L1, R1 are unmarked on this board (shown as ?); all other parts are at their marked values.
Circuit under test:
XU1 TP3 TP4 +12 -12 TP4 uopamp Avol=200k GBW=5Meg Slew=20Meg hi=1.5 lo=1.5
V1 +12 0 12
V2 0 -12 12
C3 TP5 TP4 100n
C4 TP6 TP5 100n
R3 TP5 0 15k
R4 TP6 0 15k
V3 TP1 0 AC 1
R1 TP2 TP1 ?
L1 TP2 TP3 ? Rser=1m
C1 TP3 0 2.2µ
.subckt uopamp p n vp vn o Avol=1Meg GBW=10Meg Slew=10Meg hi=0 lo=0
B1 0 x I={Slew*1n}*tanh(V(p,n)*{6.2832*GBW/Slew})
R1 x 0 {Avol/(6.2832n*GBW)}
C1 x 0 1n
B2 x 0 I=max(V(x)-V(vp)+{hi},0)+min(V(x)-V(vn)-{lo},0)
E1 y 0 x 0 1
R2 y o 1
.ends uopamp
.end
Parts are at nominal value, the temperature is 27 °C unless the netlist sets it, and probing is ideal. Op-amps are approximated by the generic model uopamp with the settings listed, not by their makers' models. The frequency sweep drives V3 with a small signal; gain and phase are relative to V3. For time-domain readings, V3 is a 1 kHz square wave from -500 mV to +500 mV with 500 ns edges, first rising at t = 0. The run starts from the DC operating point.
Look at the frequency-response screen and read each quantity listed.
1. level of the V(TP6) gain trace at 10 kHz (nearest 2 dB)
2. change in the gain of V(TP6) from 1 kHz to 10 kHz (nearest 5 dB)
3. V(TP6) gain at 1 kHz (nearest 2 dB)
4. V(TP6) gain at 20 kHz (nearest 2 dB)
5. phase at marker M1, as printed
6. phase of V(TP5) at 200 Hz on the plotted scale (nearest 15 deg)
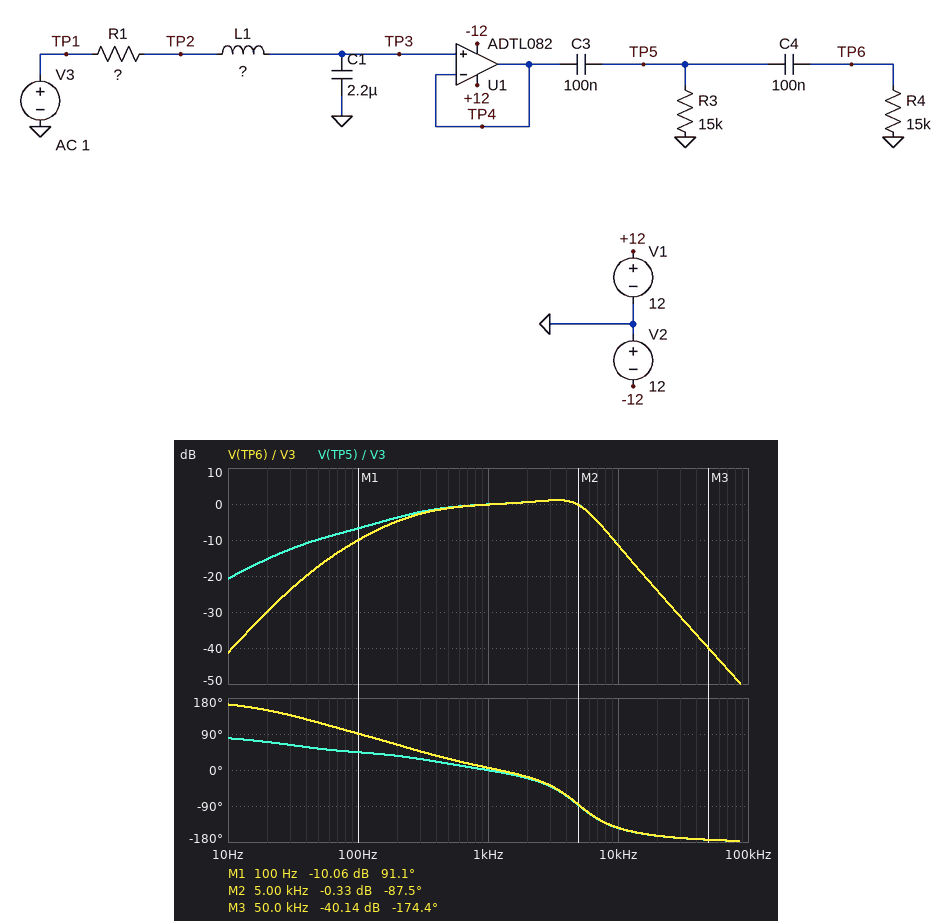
-12 dB
-10 dB
0 dB
-24 dB
91.1 deg
30 deg
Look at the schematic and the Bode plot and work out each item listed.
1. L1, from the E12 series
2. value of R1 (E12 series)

470 µH
15 Ω
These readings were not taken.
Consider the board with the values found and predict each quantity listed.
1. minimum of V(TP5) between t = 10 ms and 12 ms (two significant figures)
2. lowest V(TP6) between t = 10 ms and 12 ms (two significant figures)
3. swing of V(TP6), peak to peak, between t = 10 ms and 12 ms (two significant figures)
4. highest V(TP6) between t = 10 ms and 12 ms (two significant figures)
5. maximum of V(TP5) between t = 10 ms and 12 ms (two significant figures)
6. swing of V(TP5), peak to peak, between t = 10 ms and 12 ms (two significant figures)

-740 mV
-800 mV
1.6 V
790 mV
760 mV
1.5 V
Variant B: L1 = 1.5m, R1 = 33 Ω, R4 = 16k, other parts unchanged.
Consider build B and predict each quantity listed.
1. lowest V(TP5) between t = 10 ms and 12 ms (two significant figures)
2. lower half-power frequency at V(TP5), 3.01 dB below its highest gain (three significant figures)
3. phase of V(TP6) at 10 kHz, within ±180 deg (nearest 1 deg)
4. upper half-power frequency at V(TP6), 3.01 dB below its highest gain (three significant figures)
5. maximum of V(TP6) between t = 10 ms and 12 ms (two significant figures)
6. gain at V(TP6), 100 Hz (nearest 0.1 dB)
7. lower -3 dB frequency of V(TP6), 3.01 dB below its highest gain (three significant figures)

-620 mV
234 Hz
-158 deg
3.05 kHz
640 mV
-9.7 dB
271 Hz
